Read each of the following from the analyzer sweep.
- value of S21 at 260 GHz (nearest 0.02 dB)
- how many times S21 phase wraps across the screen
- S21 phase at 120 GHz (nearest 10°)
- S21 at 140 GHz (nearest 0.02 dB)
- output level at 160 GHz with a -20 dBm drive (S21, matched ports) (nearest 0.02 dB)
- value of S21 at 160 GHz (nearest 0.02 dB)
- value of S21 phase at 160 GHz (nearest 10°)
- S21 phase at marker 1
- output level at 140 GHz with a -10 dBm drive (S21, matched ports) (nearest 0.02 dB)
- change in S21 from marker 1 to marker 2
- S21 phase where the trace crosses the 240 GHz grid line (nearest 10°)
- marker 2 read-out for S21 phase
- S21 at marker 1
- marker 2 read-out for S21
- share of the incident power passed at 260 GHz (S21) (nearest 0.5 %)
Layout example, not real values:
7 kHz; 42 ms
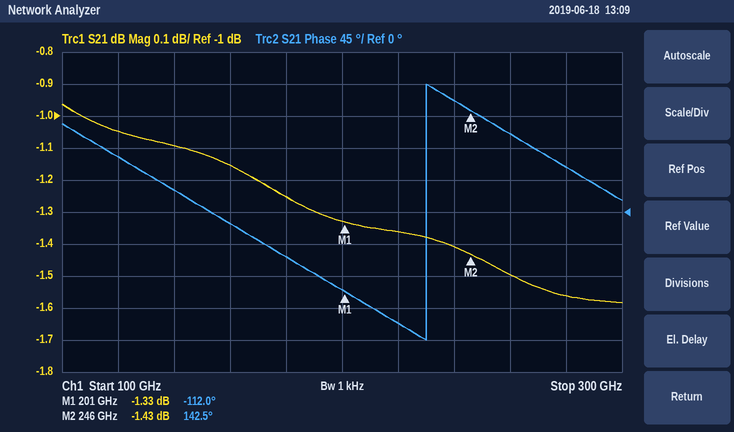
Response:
-1.50 dB; 1; 80°; -1.10 dB; -21.16 dBm; -1.16 dB; -20°; -112.0°; -11.10 dBm; -0.10 dB; 160°; 142.5°; -1.33 dB; -1.43 dB; 71.0 %
